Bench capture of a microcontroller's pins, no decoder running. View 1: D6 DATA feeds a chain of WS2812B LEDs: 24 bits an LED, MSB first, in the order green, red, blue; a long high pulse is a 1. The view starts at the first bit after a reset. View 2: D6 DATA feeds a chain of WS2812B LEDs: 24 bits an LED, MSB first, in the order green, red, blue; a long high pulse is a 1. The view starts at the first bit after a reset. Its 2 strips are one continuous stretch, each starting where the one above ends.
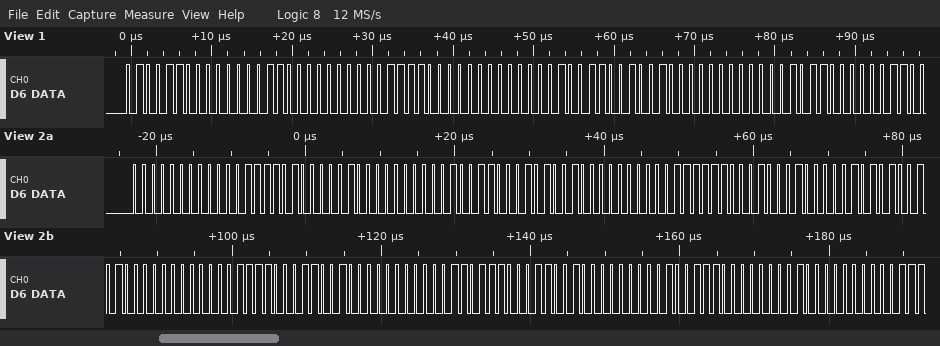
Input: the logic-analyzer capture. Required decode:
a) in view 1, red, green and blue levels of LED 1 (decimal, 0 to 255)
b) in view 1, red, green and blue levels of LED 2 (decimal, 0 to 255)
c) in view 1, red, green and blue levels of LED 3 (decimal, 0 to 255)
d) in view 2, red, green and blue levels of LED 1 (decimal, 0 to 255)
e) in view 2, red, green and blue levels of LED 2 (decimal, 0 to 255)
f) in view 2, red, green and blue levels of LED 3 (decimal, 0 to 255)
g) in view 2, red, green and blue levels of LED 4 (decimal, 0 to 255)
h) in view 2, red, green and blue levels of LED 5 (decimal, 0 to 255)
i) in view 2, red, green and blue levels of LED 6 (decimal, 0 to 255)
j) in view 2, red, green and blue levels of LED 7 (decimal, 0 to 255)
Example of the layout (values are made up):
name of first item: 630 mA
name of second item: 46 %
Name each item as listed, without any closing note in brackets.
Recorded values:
in view 1, red, green and blue levels of LED 1: 3, 76, 0
in view 1, red, green and blue levels of LED 2: 0, 60, 19
in view 1, red, green and blue levels of LED 3: 0, 36, 44
in view 2, red, green and blue levels of LED 1: 15, 0, 65
in view 2, red, green and blue levels of LED 2: 38, 0, 41
in view 2, red, green and blue levels of LED 3: 63, 0, 17
in view 2, red, green and blue levels of LED 4: 74, 5, 0
in view 2, red, green and blue levels of LED 5: 50, 30, 0
in view 2, red, green and blue levels of LED 6: 25, 55, 0
in view 2, red, green and blue levels of LED 7: 1, 78, 0
